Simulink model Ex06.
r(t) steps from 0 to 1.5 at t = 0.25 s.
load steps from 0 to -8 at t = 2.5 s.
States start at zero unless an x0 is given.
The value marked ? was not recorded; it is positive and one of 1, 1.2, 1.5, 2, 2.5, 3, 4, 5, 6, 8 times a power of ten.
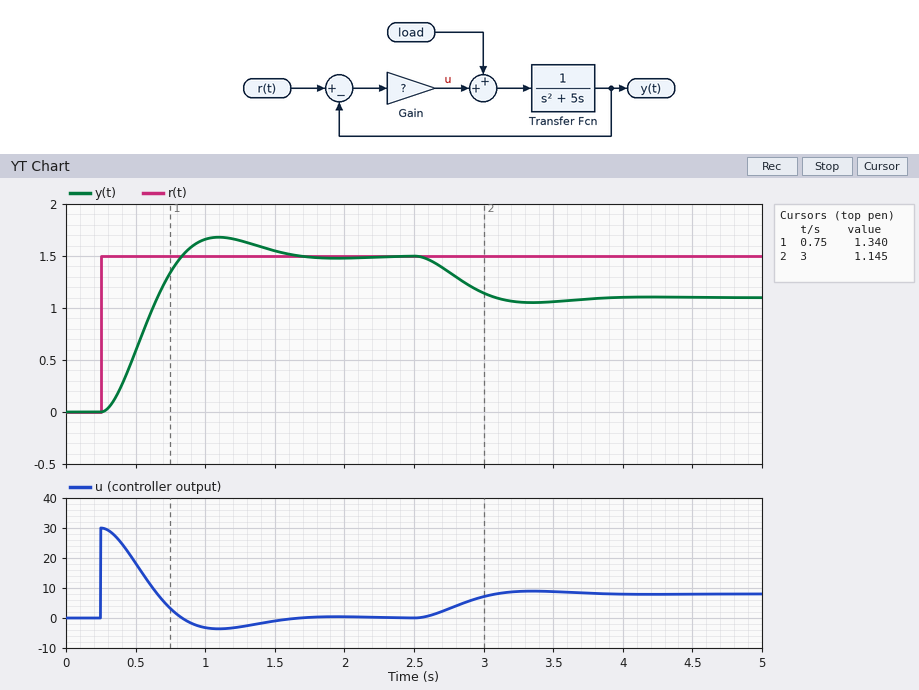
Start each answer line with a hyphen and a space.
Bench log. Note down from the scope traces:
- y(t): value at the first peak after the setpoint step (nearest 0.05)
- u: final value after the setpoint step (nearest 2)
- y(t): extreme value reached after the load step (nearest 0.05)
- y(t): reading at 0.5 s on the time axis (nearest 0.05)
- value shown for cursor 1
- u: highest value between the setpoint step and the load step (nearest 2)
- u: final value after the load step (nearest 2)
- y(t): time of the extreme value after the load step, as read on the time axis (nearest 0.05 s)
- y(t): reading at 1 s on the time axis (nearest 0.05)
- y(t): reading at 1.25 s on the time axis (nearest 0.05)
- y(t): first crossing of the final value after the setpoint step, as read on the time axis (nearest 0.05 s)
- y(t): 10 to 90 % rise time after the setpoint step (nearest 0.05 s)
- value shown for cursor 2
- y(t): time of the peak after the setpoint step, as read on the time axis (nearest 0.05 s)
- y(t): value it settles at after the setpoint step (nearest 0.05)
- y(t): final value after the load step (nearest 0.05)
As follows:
- 1.70
- 0
- 1.05
- 0.60
- 1.340
- 30
- 8
- 3.35 s
- 1.65
- 1.65
- 0.85 s
- 0.40 s
- 1.145
- 1.10 s
- 1.50
- 1.10
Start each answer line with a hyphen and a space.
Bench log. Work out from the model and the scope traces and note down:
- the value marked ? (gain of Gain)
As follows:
- 20
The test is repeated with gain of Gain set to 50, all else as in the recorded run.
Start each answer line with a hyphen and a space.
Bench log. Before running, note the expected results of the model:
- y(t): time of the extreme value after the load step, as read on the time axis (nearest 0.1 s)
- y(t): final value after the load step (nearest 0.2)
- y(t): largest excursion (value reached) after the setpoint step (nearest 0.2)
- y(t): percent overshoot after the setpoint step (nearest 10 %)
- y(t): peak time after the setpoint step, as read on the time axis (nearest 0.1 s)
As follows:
- 3.0 s
- 1.4
- 2.0
- 30 %
- 0.7 s
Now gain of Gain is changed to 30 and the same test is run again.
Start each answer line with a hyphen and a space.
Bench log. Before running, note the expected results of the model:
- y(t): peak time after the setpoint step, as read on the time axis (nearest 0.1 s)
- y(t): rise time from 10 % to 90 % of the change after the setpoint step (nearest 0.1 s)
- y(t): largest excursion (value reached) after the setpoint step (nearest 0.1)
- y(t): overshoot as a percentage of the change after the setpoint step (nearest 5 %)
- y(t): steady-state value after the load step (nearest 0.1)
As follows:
- 0.9 s
- 0.3 s
- 1.8
- 20 %
- 1.2
